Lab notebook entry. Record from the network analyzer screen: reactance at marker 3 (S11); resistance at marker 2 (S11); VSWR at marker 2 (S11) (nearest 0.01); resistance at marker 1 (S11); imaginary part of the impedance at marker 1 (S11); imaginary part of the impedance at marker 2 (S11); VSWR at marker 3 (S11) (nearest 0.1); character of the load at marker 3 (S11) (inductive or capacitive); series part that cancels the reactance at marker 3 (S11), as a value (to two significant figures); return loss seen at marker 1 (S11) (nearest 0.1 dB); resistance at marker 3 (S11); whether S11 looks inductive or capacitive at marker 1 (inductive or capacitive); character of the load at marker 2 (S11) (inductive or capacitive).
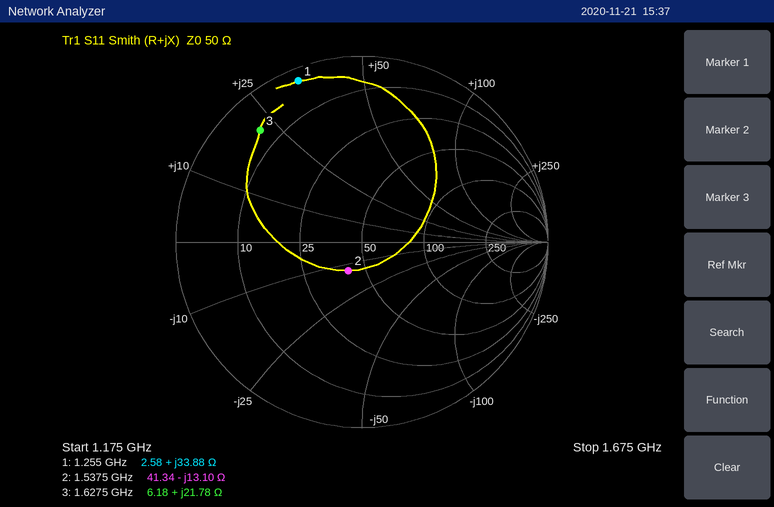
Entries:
+21.78 Ω
41.34 Ω
1.41
2.58 Ω
+33.88 Ω
-13.10 Ω
9.6
inductive
4.5 pF
0.6 dB
6.18 Ω
inductive
capacitive
